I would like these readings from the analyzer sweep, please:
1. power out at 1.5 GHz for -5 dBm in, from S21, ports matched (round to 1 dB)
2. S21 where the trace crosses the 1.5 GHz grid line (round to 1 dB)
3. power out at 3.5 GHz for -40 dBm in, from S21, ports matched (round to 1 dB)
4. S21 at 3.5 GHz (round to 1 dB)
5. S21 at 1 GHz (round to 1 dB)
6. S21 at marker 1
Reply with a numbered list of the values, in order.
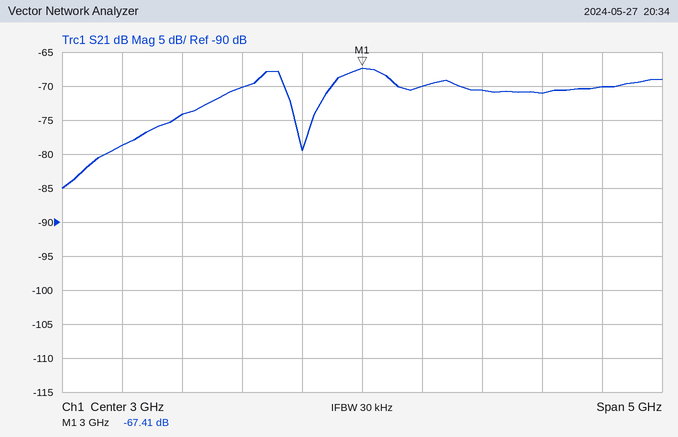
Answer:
1. -79 dBm
2. -74 dB
3. -110 dBm
4. -70 dB
5. -79 dB
6. -67.41 dB
